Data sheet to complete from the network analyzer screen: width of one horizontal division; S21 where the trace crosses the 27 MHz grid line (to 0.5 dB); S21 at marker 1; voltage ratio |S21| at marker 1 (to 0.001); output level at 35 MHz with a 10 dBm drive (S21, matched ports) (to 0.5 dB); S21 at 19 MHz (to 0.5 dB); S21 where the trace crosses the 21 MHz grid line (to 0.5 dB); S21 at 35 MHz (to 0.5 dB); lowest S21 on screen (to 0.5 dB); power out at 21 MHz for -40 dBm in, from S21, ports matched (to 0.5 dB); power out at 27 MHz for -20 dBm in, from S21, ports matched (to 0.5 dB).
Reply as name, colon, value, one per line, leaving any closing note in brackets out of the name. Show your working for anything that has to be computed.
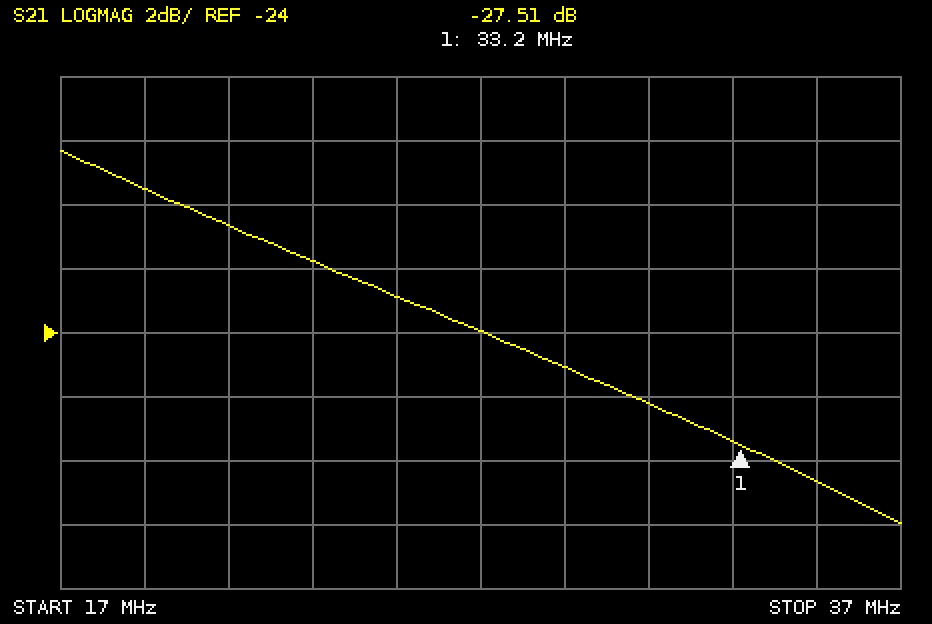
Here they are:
width of one horizontal division: 2 MHz
S21 where the trace crosses the 27 MHz grid line: -24.0 dB
S21 at marker 1: -27.51 dB
voltage ratio |S21| at marker 1: 10^(-27.51/20) ≈ 0.042
output level at 35 MHz with a 10 dBm drive (S21, matched ports): 10 dBm + (-28.5 dB) = -18.5 dBm
S21 at 19 MHz: -19.5 dB
S21 where the trace crosses the 21 MHz grid line: -20.5 dB
S21 at 35 MHz: -28.5 dB
lowest S21 on screen: -30.0 dB
power out at 21 MHz for -40 dBm in, from S21, ports matched: -40 dBm + (-20.5 dB) = -60.5 dBm
power out at 27 MHz for -20 dBm in, from S21, ports matched: -20 dBm + (-24.0 dB) = -44.0 dBm
